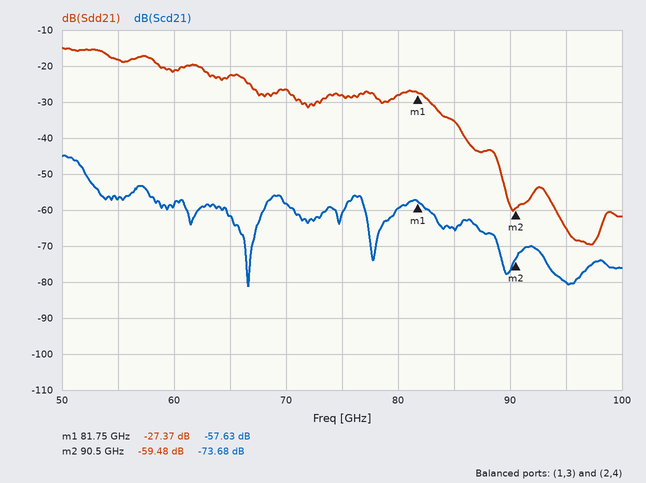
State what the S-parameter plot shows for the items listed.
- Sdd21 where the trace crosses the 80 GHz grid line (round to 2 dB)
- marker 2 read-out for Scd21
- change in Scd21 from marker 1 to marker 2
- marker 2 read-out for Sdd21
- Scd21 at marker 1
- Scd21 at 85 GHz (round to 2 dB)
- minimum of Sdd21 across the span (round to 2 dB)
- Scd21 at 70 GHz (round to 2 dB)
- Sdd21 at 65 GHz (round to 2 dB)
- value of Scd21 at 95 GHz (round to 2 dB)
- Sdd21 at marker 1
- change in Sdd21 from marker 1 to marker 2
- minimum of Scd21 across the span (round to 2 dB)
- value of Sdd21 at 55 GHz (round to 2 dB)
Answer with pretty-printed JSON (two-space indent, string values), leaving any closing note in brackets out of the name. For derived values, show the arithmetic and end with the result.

{
  "Sdd21 where the trace crosses the 80 GHz grid line": "-28 dB",
  "marker 2 read-out for Scd21": "-73.68 dB",
  "change in Scd21 from marker 1 to marker 2": "-73.68 − (-57.63) = -16.05 dB",
  "marker 2 read-out for Sdd21": "-59.48 dB",
  "Scd21 at marker 1": "-57.63 dB",
  "Scd21 at 85 GHz": "-66 dB",
  "minimum of Sdd21 across the span": "-70 dB",
  "Scd21 at 70 GHz": "-58 dB",
  "Sdd21 at 65 GHz": "-22 dB",
  "value of Scd21 at 95 GHz": "-80 dB",
  "Sdd21 at marker 1": "-27.37 dB",
  "change in Sdd21 from marker 1 to marker 2": "-59.48 − (-27.37) = -32.11 dB",
  "minimum of Scd21 across the span": "-82 dB",
  "value of Sdd21 at 55 GHz": "-18 dB"
}
